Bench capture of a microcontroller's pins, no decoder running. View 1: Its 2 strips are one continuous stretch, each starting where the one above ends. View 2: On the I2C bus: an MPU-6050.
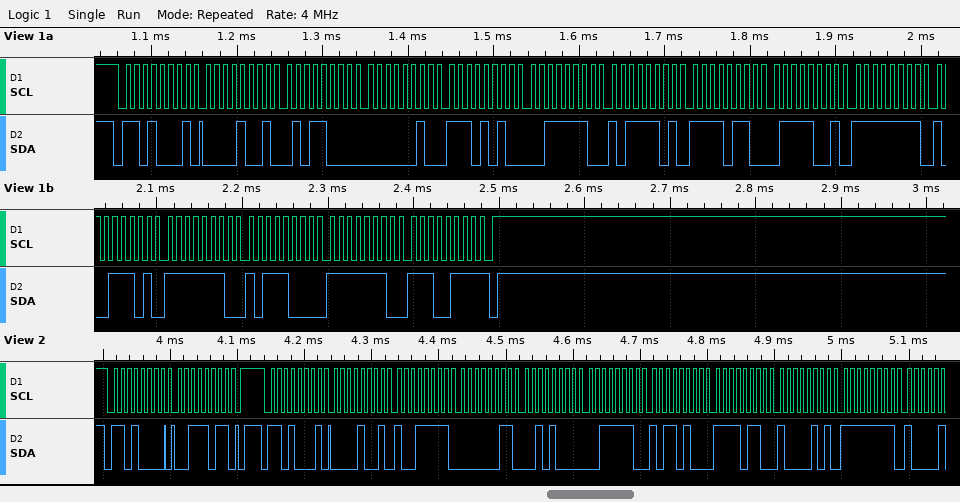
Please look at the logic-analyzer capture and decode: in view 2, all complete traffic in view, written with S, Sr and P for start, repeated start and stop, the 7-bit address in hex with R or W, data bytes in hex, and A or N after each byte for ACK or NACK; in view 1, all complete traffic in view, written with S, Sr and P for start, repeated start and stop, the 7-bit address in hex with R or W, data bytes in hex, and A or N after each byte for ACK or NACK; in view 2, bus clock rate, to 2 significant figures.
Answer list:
S 68W A 3B A P S 68R A 09 A 9F A 03 A 28 A 3E A B4 A F6 A 85 A FF A
S 68R A 09 A 58 A 02 A EA A 3E A BD A F6 A 79 A FF A 9D A FE A B8 A FE A E7 N P
100 kHz
